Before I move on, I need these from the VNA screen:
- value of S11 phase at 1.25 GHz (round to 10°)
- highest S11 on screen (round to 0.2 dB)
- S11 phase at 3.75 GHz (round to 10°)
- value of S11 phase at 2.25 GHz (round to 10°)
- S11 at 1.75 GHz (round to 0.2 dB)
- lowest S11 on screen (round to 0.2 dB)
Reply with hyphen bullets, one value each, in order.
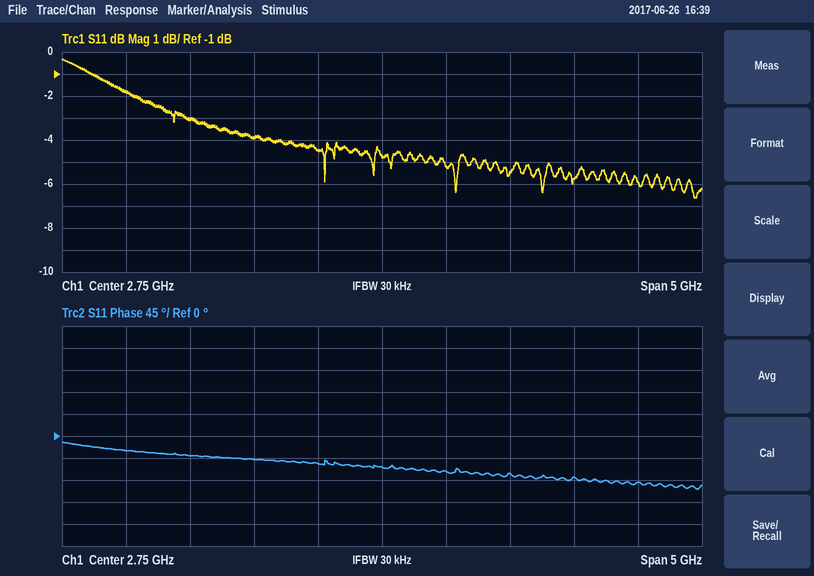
- -40°
- -0.4 dB
- -80°
- -60°
- -3.8 dB
- -6.6 dB
